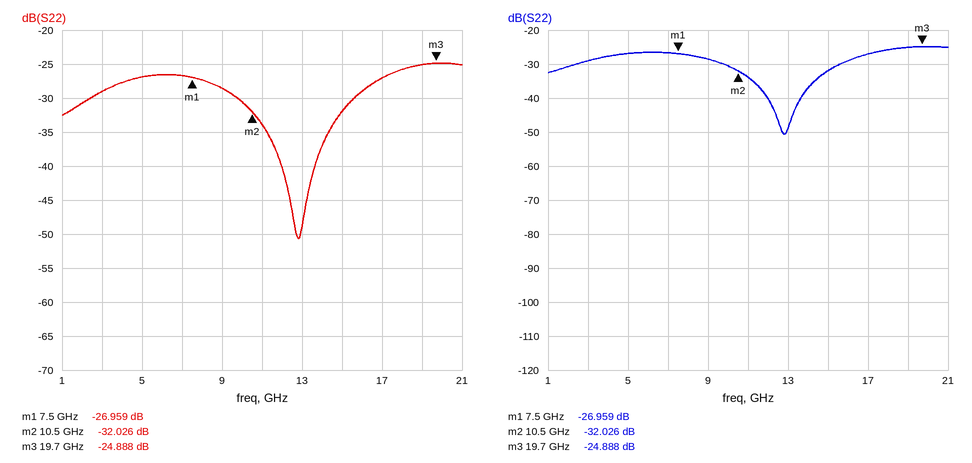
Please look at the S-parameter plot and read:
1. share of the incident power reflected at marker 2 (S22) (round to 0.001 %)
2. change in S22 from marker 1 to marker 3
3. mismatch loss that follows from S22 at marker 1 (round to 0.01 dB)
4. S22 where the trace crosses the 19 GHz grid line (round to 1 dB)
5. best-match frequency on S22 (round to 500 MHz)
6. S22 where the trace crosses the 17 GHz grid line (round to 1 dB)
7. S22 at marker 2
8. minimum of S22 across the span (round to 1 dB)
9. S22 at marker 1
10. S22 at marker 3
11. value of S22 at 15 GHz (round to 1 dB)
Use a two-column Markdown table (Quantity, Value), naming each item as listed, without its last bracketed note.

| Quantity | Value |
|---|---|
| share of the incident power reflected at marker 2 (S22) | 0.063 % |
| change in S22 from marker 1 to marker 3 | 2.071 dB |
| mismatch loss that follows from S22 at marker 1 | 0.01 dB |
| S22 where the trace crosses the 19 GHz grid line | -25 dB |
| best-match frequency on S22 | 13.0 GHz |
| S22 where the trace crosses the 17 GHz grid line | -27 dB |
| S22 at marker 2 | -32.026 dB |
| minimum of S22 across the span | -51 dB |
| S22 at marker 1 | -26.959 dB |
| S22 at marker 3 | -24.888 dB |
| value of S22 at 15 GHz | -32 dB |
